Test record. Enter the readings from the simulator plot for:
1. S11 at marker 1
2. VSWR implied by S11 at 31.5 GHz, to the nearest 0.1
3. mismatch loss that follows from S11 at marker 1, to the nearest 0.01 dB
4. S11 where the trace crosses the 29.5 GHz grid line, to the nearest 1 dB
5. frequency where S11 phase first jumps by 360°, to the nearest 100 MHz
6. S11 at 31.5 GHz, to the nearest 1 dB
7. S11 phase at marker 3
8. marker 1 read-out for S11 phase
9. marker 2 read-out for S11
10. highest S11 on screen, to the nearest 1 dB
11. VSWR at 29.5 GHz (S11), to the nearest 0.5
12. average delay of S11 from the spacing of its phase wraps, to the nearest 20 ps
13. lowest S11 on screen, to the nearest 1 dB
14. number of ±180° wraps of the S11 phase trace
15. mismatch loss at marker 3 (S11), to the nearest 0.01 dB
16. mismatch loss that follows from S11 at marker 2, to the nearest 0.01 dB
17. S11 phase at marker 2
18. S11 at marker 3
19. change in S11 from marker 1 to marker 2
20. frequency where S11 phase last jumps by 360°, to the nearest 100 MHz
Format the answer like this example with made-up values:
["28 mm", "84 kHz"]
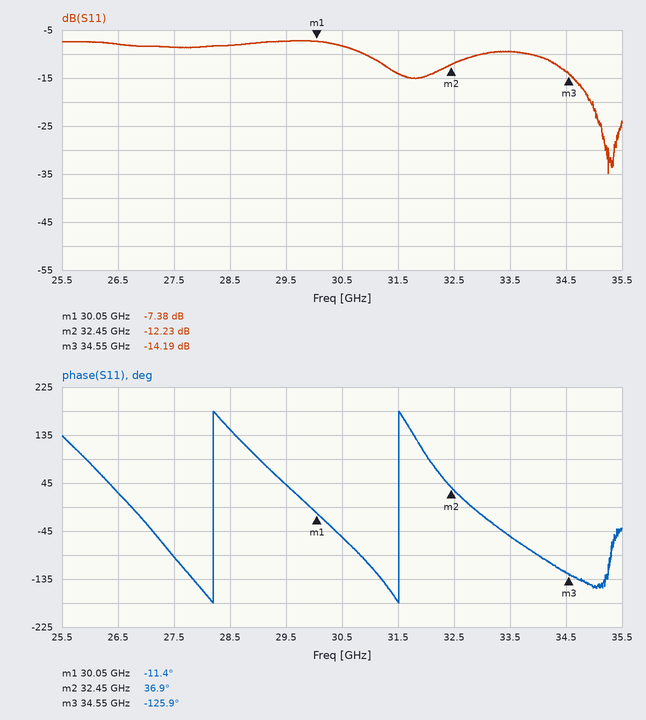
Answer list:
["-7.38 dB", "1.5", "0.88 dB", "-7 dB", "28.2 GHz", "-14 dB", "-125.9°", "-11.4°", "-12.23 dB", "-7 dB", "2.5", "300 ps", "-35 dB", "2", "0.17 dB", "0.27 dB", "36.9°", "-14.19 dB", "-4.85 dB", "31.5 GHz"]
